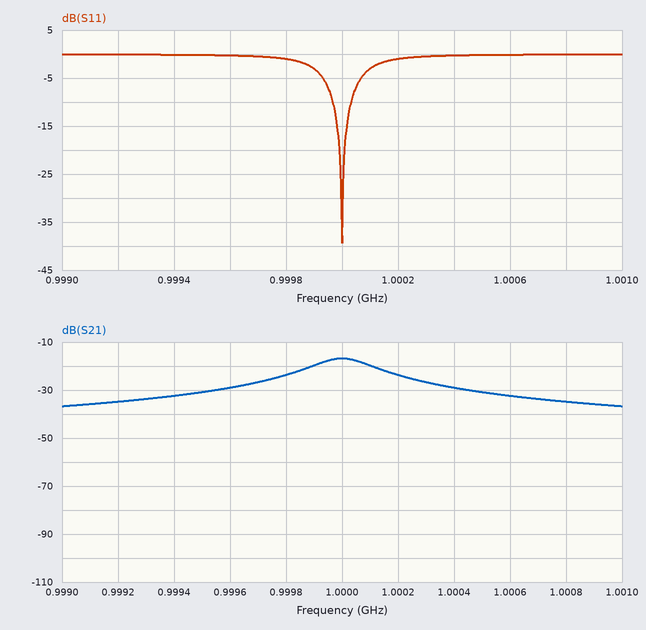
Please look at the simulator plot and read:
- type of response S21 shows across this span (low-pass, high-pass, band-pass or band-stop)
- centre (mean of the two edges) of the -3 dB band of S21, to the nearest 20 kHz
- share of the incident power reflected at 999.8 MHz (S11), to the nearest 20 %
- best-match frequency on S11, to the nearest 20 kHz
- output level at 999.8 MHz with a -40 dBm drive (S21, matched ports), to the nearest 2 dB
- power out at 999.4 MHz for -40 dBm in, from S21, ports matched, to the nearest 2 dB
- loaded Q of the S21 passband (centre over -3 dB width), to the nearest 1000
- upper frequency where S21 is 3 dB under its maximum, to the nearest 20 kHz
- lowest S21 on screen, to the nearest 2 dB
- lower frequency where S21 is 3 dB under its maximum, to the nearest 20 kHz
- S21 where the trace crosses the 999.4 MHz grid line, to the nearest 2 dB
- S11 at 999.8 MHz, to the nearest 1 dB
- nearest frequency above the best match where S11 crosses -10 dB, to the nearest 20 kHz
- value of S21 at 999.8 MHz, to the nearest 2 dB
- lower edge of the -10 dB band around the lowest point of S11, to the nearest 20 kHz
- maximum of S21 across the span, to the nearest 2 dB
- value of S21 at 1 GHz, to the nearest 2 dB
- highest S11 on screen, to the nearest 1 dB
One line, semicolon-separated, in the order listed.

band-pass; 1.00000 GHz; 80 %; 1.00000 GHz; -64 dBm; -72 dBm; 5000; 1.00010 GHz; -36 dB; 999.90 MHz; -32 dB; -1 dB; 1.00004 GHz; -24 dB; 999.96 MHz; -16 dB; -16 dB; 0 dB
